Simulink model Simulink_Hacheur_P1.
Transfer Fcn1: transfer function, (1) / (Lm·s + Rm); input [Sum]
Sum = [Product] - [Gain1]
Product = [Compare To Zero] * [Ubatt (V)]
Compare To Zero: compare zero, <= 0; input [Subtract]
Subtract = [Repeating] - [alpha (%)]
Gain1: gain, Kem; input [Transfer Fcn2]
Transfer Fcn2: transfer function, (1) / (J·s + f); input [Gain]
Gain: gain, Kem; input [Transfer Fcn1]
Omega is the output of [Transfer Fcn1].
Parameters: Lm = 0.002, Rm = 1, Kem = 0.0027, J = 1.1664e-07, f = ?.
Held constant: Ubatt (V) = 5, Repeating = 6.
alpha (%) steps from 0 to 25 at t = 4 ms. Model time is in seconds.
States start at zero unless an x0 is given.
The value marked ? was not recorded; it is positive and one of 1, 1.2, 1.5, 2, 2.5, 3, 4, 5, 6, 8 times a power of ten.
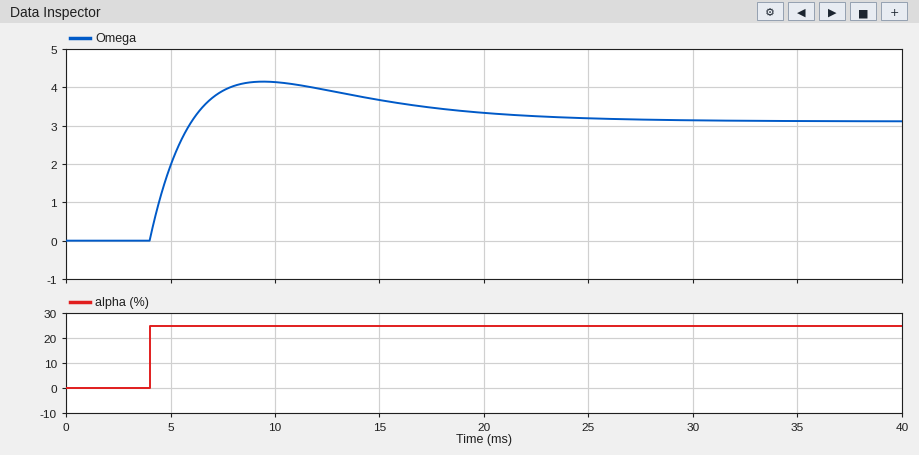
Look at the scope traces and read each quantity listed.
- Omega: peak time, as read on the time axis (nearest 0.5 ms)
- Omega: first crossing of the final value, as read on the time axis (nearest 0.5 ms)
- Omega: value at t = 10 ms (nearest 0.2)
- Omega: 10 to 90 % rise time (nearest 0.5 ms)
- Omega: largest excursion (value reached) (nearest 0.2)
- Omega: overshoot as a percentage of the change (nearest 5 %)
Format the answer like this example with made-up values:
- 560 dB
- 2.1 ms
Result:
- 9.5 ms
- 6.0 ms
- 4.2
- 1.5 ms
- 4.2
- 35 %
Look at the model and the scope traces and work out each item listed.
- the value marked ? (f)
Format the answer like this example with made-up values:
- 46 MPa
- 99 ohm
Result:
- 1.2e-05
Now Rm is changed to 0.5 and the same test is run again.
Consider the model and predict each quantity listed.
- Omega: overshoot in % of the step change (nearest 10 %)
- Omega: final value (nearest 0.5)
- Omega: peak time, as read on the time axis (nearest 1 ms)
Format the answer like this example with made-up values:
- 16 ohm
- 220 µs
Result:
- 50 %
- 4.5
- 11 ms
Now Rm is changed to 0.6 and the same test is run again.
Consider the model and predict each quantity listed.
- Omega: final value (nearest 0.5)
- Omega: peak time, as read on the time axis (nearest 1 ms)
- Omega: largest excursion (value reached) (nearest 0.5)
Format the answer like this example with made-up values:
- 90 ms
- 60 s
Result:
- 4.0
- 11 ms
- 6.0
